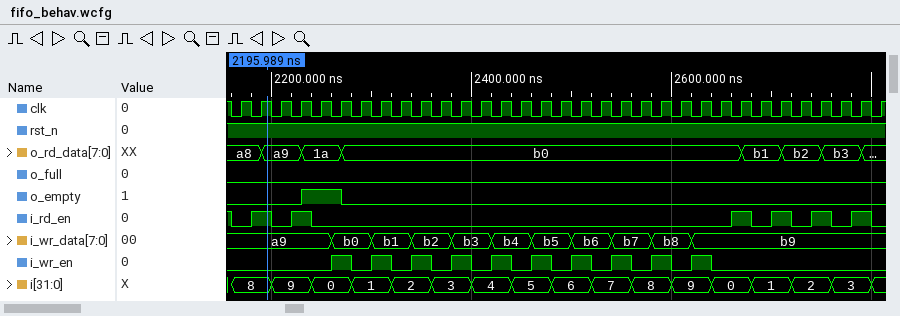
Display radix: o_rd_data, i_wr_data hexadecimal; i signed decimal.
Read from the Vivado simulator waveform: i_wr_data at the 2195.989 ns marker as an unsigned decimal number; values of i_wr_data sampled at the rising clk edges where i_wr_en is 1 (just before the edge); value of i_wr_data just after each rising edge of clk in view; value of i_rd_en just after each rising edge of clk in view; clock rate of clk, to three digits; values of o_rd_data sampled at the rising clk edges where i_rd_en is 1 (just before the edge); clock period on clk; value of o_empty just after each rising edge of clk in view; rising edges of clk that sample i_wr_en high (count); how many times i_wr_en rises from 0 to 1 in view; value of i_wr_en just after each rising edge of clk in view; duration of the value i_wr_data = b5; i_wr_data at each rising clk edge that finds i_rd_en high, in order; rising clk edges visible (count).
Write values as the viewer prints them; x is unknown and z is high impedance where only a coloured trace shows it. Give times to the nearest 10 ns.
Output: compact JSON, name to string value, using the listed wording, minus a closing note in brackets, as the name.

{"i_wr_data at the 2195.989 ns marker as an unsigned decimal number": "169", "values of i_wr_data sampled at the rising clk edges where i_wr_en is 1": "b0, b1, b2, b3, b4, b5, b6, b7, b8, b9", "value of i_wr_data just after each rising edge of clk in view": "a9, a9, a9, a9, a9, b0, b0, b1, b1, b2, b2, b3, b3, b4, b4, b5, b5, b6, b6, b7, b7, b8, b8, b9, b9, b9, b9, b9, b9, b9, b9, b9, b9", "value of i_rd_en just after each rising edge of clk in view": "0 1 0 1 0 0 0 0 0 0 0 0 0 0 0 0 0 0 0 0 0 0 0 0 0 1 0 1 0 1 0 1 0", "clock rate of clk, to three digits": "50.0 MHz", "values of o_rd_data sampled at the rising clk edges where i_rd_en is 1": "a8, a9, b0, b1, b2, b3", "clock period on clk": "20 ns", "value of o_empty just after each rising edge of clk in view": "0 0 0 1 1 0 0 0 0 0 0 0 0 0 0 0 0 0 0 0 0 0 0 0 0 0 0 0 0 0 0 0 0", "rising edges of clk that sample i_wr_en high": "10", "how many times i_wr_en rises from 0 to 1 in view": "10", "value of i_wr_en just after each rising edge of clk in view": "0 0 0 0 0 1 0 1 0 1 0 1 0 1 0 1 0 1 0 1 0 1 0 1 0 0 0 0 0 0 0 0 0", "duration of the value i_wr_data = b5": "40 ns", "i_wr_data at each rising clk edge that finds i_rd_en high, in order": "a9, a9, b9, b9, b9, b9", "rising clk edges visible": "33"}
